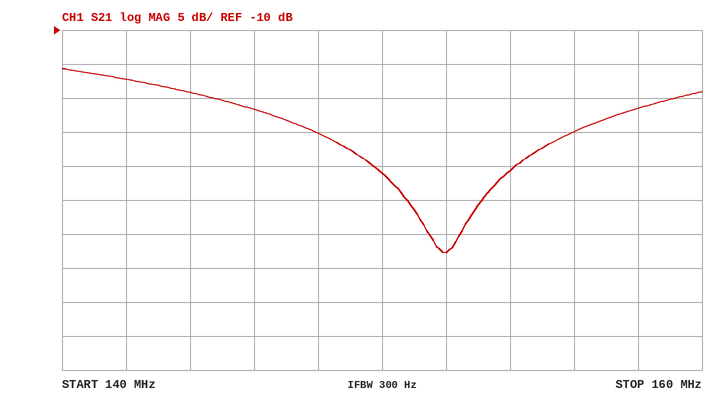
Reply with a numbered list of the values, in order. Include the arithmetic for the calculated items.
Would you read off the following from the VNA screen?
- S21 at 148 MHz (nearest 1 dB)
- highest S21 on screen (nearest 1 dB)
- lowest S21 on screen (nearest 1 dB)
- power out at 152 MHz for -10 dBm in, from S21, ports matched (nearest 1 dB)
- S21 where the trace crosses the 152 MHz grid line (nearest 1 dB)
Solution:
1. -25 dB
2. -16 dB
3. -43 dB
4. -10 dBm + (-43 dB) = -53 dBm
5. -43 dB
